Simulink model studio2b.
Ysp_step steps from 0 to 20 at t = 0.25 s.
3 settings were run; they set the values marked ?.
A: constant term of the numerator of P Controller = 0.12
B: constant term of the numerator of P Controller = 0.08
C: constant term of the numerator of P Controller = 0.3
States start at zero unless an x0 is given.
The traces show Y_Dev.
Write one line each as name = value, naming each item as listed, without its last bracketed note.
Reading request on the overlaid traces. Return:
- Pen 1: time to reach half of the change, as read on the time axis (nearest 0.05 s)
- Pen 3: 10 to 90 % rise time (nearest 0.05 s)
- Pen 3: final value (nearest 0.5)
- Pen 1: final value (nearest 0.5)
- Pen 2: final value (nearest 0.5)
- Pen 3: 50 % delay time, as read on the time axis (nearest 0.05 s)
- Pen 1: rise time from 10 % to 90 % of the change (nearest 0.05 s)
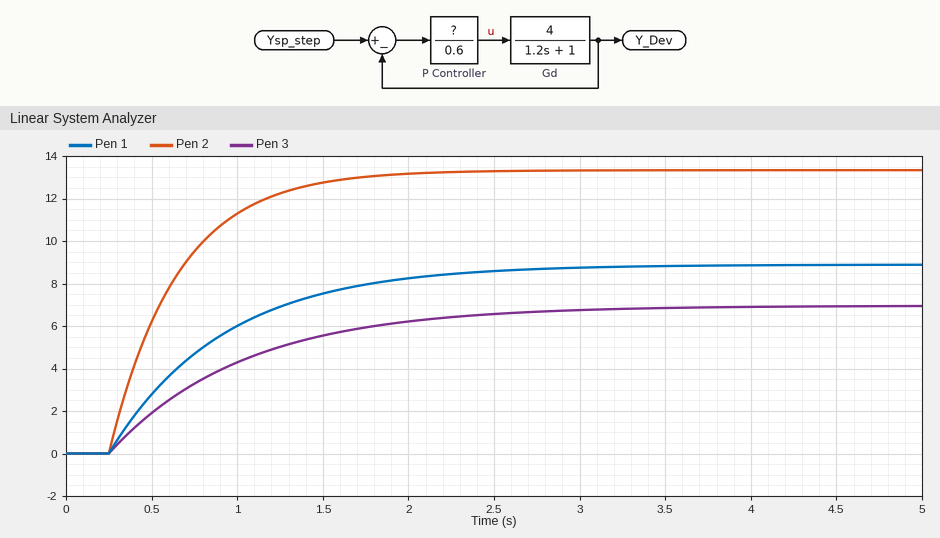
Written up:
Pen 1: time to reach half of the change, as read on the time axis = 0.70 s
Pen 3: 10 to 90 % rise time = 1.70 s
Pen 3: final value = 7.0
Pen 1: final value = 9.0
Pen 2: final value = 13.5
Pen 3: 50 % delay time, as read on the time axis = 0.80 s
Pen 1: rise time from 10 % to 90 % of the change = 1.45 s
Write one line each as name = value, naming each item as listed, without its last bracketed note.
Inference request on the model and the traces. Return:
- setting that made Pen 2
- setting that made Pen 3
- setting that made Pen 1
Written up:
setting that made Pen 2 = C
setting that made Pen 3 = B
setting that made Pen 1 = A
